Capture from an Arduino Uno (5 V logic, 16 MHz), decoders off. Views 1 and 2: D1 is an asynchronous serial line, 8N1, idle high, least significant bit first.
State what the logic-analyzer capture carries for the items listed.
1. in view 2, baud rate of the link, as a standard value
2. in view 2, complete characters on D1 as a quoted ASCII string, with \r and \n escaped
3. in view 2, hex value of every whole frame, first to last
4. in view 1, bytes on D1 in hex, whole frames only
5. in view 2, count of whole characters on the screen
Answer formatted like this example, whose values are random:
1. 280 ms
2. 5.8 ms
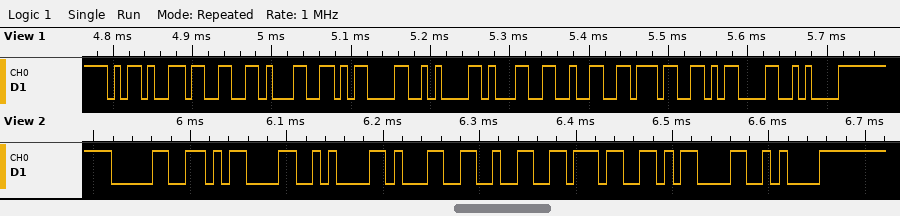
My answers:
1. 115200 baud
2. "0\r\n127\r\n"
3. 30 0D 0A 31 32 37 0D 0A
4. 2D 33 31 0D 0A 31 32 37 0D 0A
5. 8
